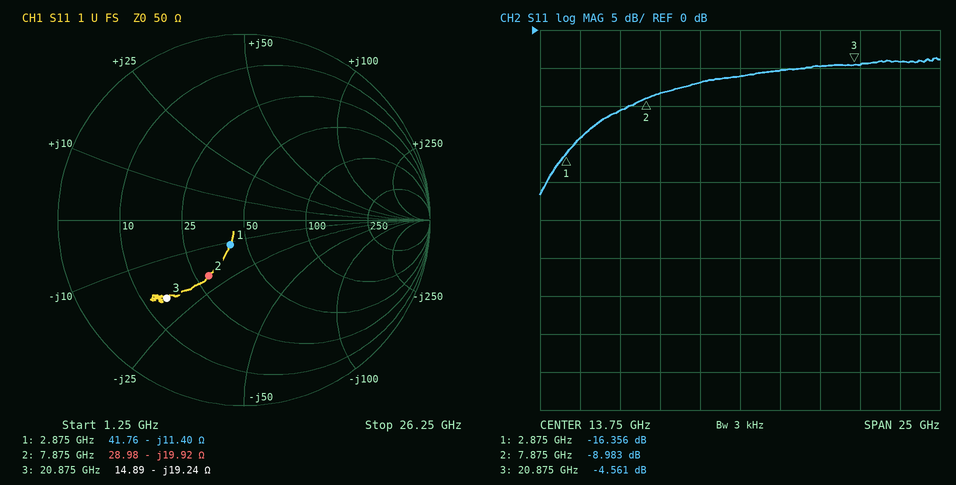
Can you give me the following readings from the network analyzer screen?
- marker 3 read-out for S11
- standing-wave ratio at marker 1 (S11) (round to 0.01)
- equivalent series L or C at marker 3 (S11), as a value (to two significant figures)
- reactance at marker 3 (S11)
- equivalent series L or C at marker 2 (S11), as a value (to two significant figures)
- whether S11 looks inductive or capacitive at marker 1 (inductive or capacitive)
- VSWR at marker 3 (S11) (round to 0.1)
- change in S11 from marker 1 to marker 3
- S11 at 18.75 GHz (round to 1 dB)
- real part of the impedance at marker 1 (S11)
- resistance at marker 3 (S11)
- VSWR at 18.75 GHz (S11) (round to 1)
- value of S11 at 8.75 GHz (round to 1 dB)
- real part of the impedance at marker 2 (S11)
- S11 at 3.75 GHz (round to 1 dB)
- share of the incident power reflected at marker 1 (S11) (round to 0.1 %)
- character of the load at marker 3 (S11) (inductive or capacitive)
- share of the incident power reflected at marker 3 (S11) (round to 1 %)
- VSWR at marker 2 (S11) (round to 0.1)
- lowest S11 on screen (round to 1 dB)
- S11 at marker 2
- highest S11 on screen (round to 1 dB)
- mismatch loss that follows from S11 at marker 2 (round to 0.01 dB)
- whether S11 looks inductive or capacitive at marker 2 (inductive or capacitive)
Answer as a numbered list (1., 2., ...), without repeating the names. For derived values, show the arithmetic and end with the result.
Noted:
1. -4.561 dB
2. 1.36
3. C = 1/(2π × 20.875 GHz × 19.24 Ω) ≈ 396 fF, so 400 fF to two significant figures
4. -19.24 Ω
5. C = 1/(2π × 7.875 GHz × 19.92 Ω) ≈ 1.0 pF
6. capacitive
7. 3.9
8. -4.561 − (-16.356) = 11.795 dB
9. -5 dB
10. 41.76 Ω
11. 14.89 Ω
12. |Γ| = 10^(-5/20) = 0.5623; VSWR = (1 + 0.5623)/(1 − 0.5623) ≈ 4
13. -8 dB
14. 28.98 Ω
15. -14 dB
16. 10^(-16.356/10) ≈ 2.3 %
17. capacitive
18. 10^(-4.561/10) ≈ 35 %
19. 2.1
20. -22 dB
21. -8.983 dB
22. -4 dB
23. −10 log10(1 − 10^(-8.983/10)) ≈ 0.59 dB
24. capacitive
